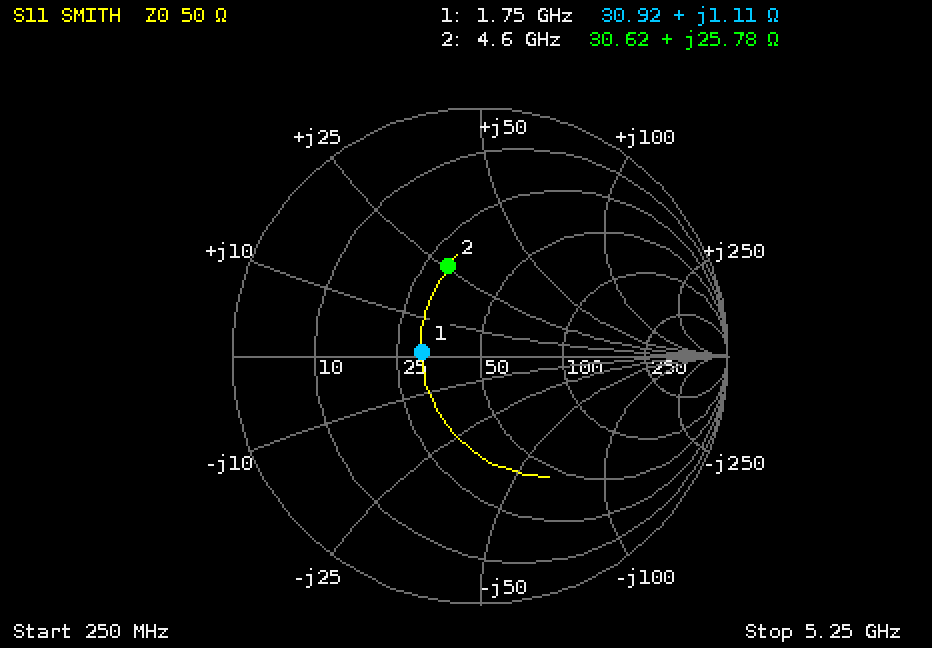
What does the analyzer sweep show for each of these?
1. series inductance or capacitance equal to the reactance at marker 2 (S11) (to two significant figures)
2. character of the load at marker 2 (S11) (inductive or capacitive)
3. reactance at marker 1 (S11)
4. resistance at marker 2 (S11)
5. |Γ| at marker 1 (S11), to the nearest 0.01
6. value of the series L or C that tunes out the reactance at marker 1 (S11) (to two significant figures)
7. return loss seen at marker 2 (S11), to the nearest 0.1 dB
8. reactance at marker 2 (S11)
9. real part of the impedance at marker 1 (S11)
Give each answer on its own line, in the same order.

890 pH
inductive
+1.11 Ω
30.62 Ω
0.24
82 pF
8.4 dB
+25.78 Ω
30.92 Ω
